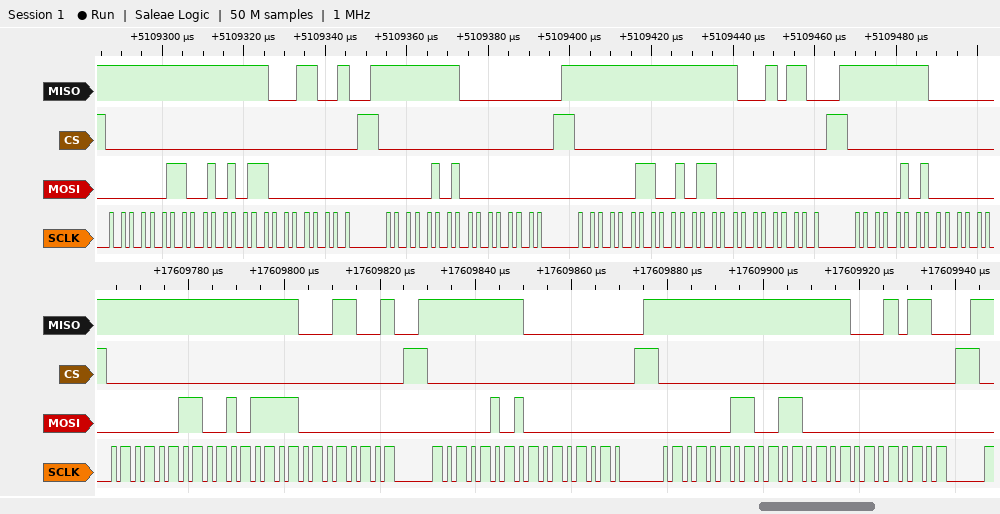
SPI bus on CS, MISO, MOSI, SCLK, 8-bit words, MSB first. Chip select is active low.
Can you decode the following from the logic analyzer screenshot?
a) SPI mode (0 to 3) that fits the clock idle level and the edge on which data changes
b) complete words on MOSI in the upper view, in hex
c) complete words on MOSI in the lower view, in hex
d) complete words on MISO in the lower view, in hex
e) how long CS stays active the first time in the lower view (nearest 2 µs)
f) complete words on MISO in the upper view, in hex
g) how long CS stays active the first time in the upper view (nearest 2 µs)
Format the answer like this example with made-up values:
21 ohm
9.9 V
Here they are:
0
03, 2B, 00, 05, 00, 03, 2C, 00, 05
03, 2F, 00, 05, 00, 03, 30, 00
FF, FF, 19, FF, 00, FF, FF, 16
62 µs
FF, FF, 19, FF, 00, FF, FF, 16, FF
62 µs
